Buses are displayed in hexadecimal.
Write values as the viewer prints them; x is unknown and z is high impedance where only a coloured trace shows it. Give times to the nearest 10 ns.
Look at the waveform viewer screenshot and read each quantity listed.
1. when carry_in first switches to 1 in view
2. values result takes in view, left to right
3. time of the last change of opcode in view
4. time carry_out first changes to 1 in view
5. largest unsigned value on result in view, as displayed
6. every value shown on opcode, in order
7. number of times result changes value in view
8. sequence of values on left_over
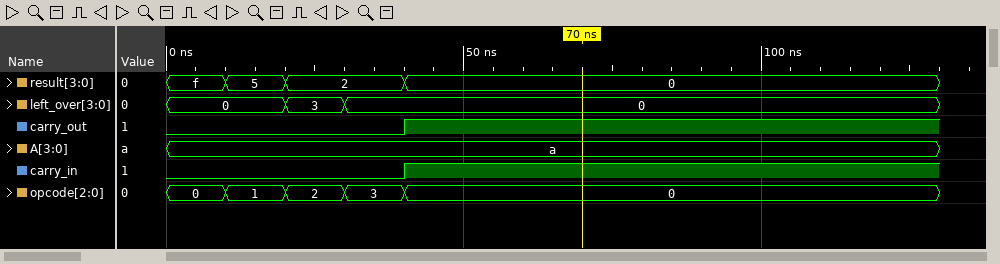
40 ns
f, 5, 2, 0
40 ns
40 ns
f
0, 1, 2, 3, 0
3
0, 3, 0
